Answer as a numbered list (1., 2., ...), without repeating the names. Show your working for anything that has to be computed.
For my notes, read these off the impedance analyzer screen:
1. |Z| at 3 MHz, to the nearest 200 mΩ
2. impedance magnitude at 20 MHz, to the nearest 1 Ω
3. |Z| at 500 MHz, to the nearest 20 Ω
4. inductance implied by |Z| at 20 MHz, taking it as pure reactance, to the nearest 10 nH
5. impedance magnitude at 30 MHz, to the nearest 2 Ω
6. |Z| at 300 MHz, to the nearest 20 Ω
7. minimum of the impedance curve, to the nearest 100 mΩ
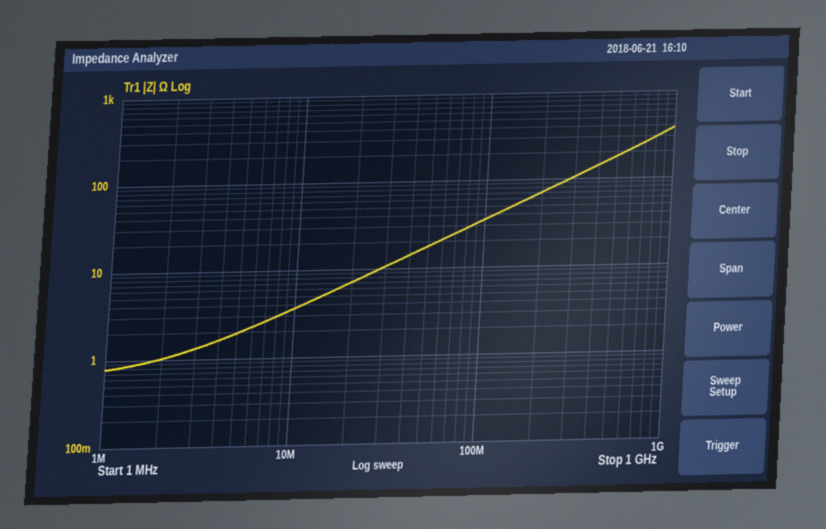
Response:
1. 1.4 Ω
2. 7 Ω
3. 180 Ω
4. L = 7 Ω/(2π × 20 MHz) ≈ 55.7 nH, so 60 nH to the nearest 10 nH
5. 10 Ω
6. 100 Ω
7. 800 mΩ
